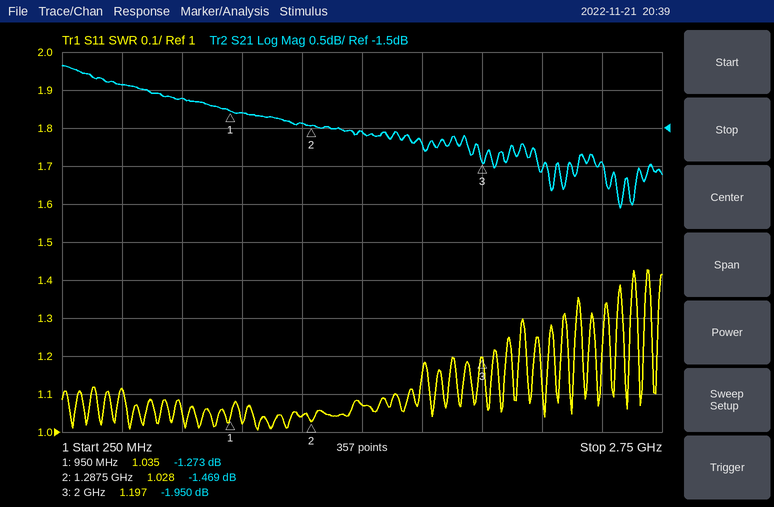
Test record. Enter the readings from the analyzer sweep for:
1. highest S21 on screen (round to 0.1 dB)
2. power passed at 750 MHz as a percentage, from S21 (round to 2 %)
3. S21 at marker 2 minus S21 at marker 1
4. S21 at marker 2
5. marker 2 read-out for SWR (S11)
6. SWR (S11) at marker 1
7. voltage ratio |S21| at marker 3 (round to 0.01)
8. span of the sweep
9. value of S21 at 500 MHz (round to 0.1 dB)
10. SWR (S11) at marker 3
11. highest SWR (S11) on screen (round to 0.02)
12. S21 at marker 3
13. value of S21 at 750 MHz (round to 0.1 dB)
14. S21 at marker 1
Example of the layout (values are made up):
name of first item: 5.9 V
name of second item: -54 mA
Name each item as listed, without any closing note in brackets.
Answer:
highest S21 on screen: -0.7 dB
power passed at 750 MHz as a percentage, from S21: 78 %
S21 at marker 2 minus S21 at marker 1: -0.196 dB
S21 at marker 2: -1.469 dB
marker 2 read-out for SWR: 1.028
SWR (S11) at marker 1: 1.035
voltage ratio |S21| at marker 3: 0.80
span of the sweep: 2.5 GHz
value of S21 at 500 MHz: -0.9 dB
SWR (S11) at marker 3: 1.197
highest SWR (S11) on screen: 1.42
S21 at marker 3: -1.950 dB
value of S21 at 750 MHz: -1.1 dB
S21 at marker 1: -1.273 dB
